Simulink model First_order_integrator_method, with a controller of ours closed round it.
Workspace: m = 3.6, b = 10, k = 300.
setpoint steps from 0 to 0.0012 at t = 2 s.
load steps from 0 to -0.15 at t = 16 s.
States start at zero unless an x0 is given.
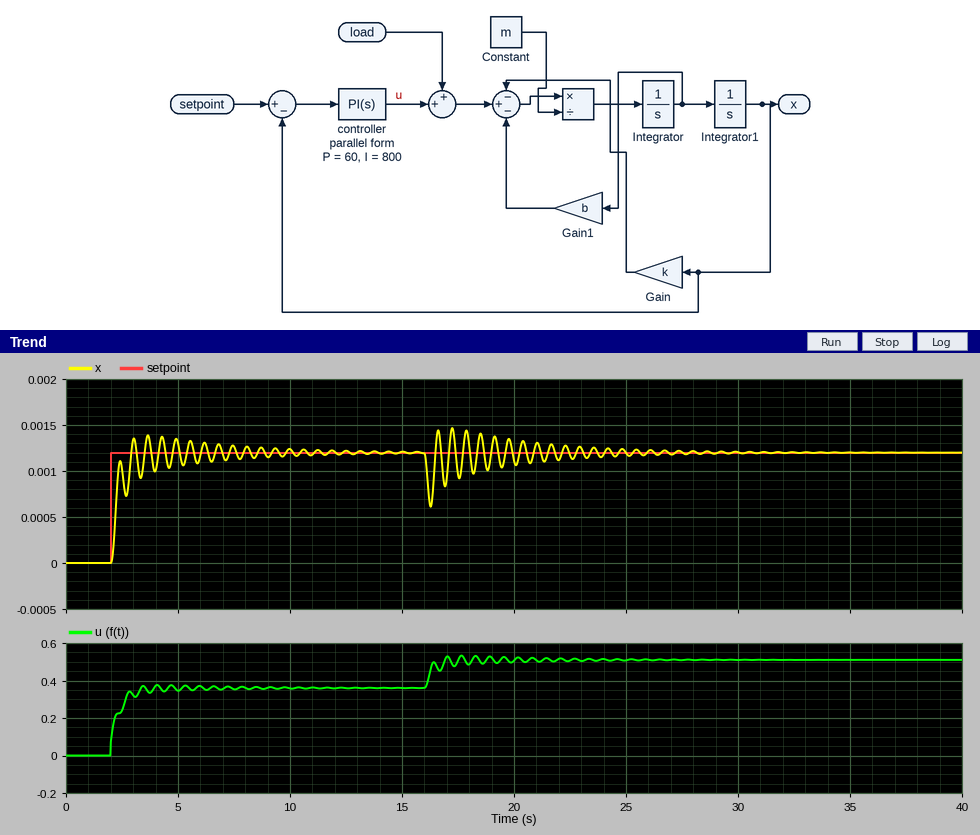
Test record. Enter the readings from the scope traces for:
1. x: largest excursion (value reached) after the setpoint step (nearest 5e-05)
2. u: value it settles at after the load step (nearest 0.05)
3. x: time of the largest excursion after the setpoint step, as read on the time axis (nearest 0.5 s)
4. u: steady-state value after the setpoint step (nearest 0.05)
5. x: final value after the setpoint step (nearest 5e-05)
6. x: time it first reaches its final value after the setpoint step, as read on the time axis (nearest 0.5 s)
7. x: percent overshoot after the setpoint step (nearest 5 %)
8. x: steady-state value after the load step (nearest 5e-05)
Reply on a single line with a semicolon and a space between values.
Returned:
0.00140; 0.50; 3.5 s; 0.35; 0.00120; 3.0 s; 15 %; 0.00120
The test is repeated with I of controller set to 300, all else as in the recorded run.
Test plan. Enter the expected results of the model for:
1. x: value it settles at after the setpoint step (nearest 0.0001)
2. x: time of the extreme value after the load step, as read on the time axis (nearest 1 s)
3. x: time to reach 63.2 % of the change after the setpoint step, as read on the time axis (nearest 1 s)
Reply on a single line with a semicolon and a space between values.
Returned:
0.0012; 16 s; 3 s
